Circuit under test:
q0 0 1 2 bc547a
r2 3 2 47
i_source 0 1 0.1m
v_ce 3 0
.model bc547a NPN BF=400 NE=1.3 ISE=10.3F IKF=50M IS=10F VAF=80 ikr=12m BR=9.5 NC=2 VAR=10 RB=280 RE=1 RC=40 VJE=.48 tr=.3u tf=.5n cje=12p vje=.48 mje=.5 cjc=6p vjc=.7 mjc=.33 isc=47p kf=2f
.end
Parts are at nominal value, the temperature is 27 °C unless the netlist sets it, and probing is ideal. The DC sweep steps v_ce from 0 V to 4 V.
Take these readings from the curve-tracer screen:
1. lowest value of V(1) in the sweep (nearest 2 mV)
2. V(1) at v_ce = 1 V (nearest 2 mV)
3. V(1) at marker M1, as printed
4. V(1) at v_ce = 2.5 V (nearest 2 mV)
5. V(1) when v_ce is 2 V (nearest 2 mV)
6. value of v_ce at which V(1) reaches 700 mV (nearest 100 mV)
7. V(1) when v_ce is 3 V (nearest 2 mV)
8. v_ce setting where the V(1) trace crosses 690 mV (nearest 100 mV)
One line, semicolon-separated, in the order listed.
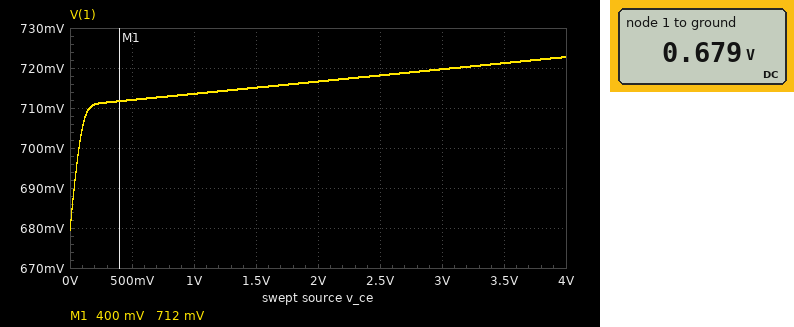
680 mV; 714 mV; 712 mV; 718 mV; 716 mV; 100 mV; 720 mV; 0 V
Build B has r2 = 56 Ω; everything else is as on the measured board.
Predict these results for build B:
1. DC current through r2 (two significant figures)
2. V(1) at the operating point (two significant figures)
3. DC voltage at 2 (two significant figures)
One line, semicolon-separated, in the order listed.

31 µA; 680 mV; 1.7 mV
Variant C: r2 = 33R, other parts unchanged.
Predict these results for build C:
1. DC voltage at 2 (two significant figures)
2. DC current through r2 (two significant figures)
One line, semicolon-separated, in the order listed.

1.2 mV; 37 µA
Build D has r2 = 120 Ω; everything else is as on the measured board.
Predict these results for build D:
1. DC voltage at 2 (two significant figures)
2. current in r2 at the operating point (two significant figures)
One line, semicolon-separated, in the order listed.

2.5 mV; 21 µA
